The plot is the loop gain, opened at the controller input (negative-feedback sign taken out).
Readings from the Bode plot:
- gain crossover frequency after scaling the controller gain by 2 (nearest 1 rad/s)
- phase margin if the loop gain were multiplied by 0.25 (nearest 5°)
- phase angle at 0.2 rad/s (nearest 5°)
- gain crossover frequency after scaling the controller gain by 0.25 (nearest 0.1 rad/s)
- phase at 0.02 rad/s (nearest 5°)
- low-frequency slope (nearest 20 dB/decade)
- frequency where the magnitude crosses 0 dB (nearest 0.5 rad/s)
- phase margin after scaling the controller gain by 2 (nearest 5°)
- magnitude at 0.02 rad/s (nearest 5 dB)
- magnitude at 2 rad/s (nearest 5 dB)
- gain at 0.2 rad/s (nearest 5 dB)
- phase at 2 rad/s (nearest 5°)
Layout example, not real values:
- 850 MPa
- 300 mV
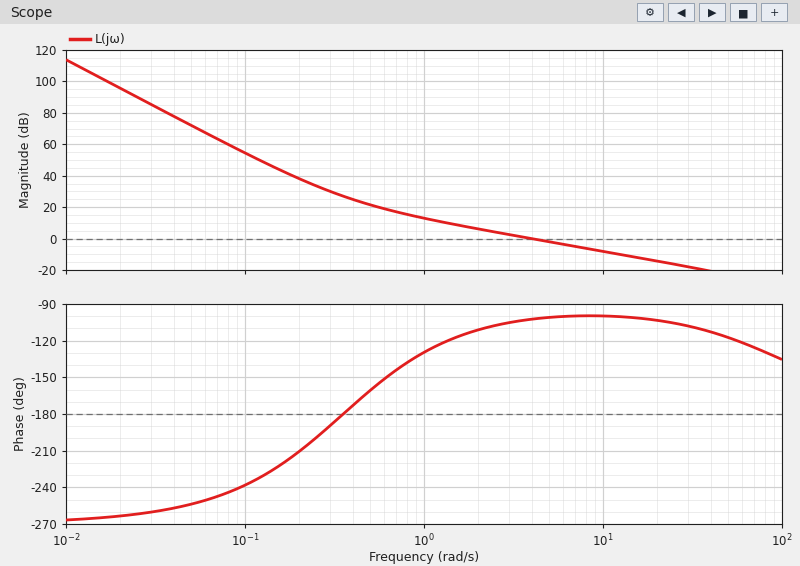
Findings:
- 8 rad/s
- 55°
- -210°
- 1.1 rad/s
- -265°
- -60 dB/decade
- 4.0 rad/s
- 80°
- 95 dB
- 5 dB
- 40 dB
- -110°
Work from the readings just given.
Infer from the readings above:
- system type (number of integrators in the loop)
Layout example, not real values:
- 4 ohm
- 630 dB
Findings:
- 3
